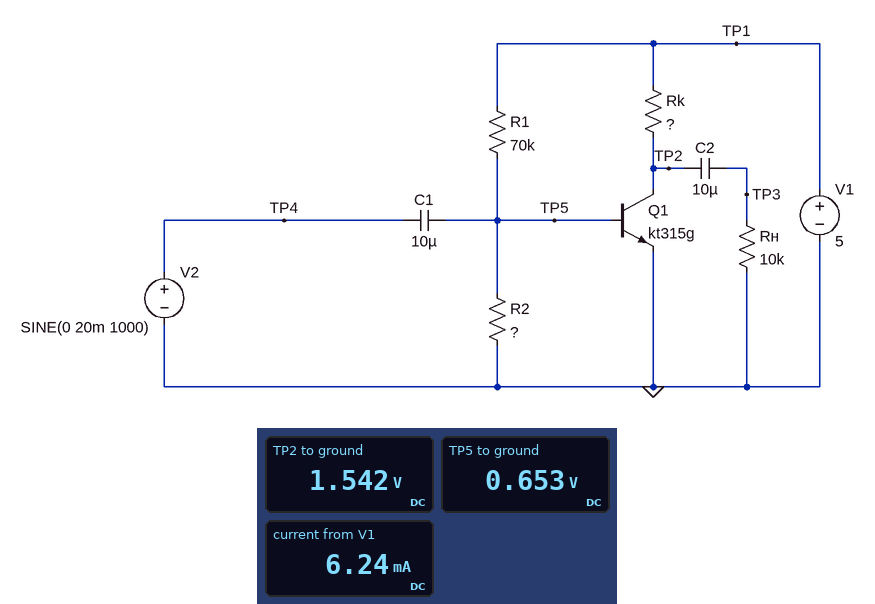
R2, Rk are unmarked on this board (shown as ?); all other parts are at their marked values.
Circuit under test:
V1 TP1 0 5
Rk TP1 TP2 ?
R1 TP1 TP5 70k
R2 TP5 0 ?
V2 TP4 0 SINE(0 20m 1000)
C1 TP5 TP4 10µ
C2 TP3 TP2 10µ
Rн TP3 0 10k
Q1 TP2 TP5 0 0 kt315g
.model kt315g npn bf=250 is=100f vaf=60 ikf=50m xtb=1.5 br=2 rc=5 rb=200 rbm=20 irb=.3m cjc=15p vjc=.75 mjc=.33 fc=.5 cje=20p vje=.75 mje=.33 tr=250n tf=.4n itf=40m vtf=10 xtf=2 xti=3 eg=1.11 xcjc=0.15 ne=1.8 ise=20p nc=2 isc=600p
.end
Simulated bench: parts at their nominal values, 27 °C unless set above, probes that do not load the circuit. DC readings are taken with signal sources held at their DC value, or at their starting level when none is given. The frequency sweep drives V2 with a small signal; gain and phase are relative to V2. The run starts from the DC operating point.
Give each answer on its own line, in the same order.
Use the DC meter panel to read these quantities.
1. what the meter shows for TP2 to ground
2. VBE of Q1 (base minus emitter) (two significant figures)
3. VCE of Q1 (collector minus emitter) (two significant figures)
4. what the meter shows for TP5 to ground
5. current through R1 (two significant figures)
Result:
1.542 V
650 mV
1.5 V
0.653 V
62 µA
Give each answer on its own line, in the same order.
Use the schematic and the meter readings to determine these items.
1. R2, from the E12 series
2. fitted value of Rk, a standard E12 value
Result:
47 kΩ
560 Ω
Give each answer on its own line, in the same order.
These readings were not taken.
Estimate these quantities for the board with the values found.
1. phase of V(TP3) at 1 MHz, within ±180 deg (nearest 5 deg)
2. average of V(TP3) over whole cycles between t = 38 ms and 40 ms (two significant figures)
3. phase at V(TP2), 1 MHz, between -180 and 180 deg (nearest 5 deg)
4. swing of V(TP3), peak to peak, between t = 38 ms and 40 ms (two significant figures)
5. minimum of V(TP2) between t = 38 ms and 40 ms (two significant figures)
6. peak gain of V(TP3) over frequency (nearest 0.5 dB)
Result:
165 deg
150 mV
165 deg
3.0 V
200 mV
39.0 dB
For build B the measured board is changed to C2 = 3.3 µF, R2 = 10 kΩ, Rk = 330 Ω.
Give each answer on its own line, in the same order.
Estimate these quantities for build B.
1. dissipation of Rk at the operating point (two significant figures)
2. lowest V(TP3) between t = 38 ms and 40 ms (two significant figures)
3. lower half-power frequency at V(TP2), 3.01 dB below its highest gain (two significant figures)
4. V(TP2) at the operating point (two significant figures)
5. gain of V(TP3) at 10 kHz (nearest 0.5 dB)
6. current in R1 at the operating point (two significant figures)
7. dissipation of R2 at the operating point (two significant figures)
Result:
60 µW
-130 mV
4.1 Hz
4.9 V
14.0 dB
63 µA
33 µW
